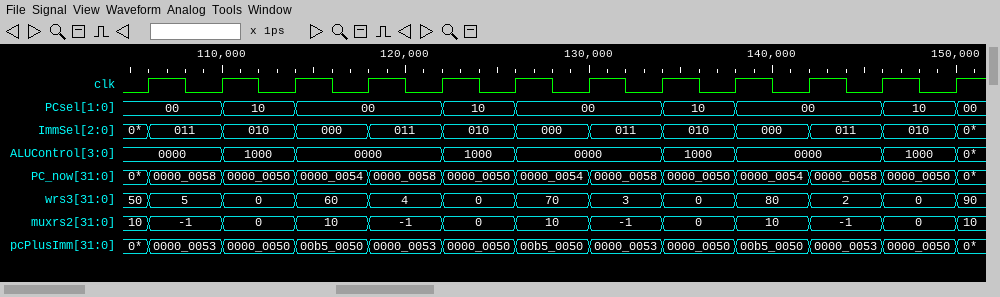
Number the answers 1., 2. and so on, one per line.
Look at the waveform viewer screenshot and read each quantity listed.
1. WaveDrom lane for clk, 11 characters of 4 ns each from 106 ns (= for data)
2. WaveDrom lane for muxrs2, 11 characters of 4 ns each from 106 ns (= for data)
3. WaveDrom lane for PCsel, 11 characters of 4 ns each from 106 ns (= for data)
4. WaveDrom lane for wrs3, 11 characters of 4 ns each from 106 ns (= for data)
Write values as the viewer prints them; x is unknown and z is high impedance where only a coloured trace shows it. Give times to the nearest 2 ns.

1. {name: 'clk', wave: 'p..........'}
2. {name: 'muxrs2', wave: '===========', data: '-1 0 10 -1 0 10 -1 0 10 -1 0'}
3. {name: 'PCsel', wave: '===.==.==.=', data: '00 10 00 10 00 10 00 10'}
4. {name: 'wrs3', wave: '===========', data: '5 0 60 4 0 70 3 0 80 2 0'}
